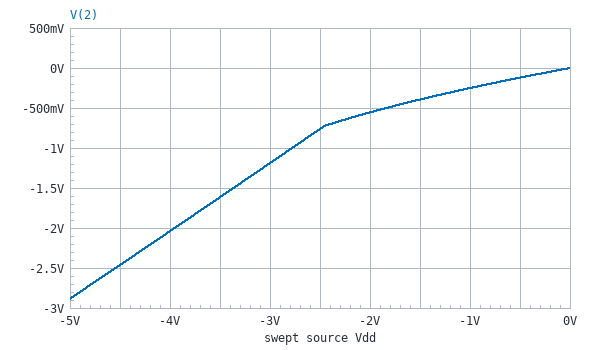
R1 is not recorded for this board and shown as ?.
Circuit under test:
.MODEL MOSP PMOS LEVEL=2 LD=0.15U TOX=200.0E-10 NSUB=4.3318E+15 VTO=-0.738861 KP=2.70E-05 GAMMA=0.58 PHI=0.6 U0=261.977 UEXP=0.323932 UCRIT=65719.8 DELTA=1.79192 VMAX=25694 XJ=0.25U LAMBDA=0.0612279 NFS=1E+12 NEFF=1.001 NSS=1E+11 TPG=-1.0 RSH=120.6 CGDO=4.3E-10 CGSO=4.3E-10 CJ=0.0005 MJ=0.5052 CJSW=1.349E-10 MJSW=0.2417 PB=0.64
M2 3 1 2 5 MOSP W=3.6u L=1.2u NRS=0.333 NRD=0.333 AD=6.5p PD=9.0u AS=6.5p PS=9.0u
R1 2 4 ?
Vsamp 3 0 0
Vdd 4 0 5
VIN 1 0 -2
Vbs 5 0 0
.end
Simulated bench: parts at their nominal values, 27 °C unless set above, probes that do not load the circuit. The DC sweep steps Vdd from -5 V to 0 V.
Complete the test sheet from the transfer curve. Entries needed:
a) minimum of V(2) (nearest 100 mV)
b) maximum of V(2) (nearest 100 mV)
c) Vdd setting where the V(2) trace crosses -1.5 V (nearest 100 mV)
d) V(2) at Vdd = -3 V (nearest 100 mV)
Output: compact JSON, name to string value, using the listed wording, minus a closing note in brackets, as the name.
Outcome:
{"minimum of V(2)": "-2.9 V", "maximum of V(2)": "0 V", "Vdd setting where the V(2) trace crosses -1.5 V": "-3.4 V", "V(2) at Vdd = -3 V": "-1.2 V"}
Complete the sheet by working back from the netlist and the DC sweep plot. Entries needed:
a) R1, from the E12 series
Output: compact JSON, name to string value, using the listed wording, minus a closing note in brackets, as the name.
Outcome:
{"R1, from the E12 series": "33 kΩ"}
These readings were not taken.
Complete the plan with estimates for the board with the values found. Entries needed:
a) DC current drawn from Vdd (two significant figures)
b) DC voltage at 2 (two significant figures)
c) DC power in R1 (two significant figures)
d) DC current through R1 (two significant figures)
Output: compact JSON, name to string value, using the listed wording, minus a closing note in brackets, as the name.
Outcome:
{"DC current drawn from Vdd": "130 µA", "DC voltage at 2": "590 mV", "DC power in R1": "590 µW", "DC current through R1": "130 µA"}
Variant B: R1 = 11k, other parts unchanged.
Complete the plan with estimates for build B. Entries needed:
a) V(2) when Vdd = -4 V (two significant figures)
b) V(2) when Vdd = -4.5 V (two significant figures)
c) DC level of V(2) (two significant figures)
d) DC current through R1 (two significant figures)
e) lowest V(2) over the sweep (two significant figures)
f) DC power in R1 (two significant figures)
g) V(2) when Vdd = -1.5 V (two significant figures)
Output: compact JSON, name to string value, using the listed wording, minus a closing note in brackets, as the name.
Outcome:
{"V(2) when Vdd = -4 V": "-3.3 V", "V(2) when Vdd = -4.5 V": "-3.7 V", "DC level of V(2)": "640 mV", "DC current through R1": "400 µA", "lowest V(2) over the sweep": "-4.2 V", "DC power in R1": "1.7 mW", "V(2) when Vdd = -1.5 V": "-910 mV"}
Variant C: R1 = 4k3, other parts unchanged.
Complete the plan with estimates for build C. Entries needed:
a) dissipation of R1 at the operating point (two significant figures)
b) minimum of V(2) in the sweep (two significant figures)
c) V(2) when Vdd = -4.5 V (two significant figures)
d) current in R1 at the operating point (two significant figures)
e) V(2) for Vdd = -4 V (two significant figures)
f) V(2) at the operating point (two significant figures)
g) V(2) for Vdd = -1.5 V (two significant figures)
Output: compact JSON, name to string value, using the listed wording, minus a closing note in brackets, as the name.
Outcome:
{"dissipation of R1 at the operating point": "4.3 mW", "minimum of V(2) in the sweep": "-4.7 V", "V(2) when Vdd = -4.5 V": "-4.2 V", "current in R1 at the operating point": "1.0 mA", "V(2) for Vdd = -4 V": "-3.7 V", "V(2) at the operating point": "690 mV", "V(2) for Vdd = -1.5 V": "-1.3 V"}
